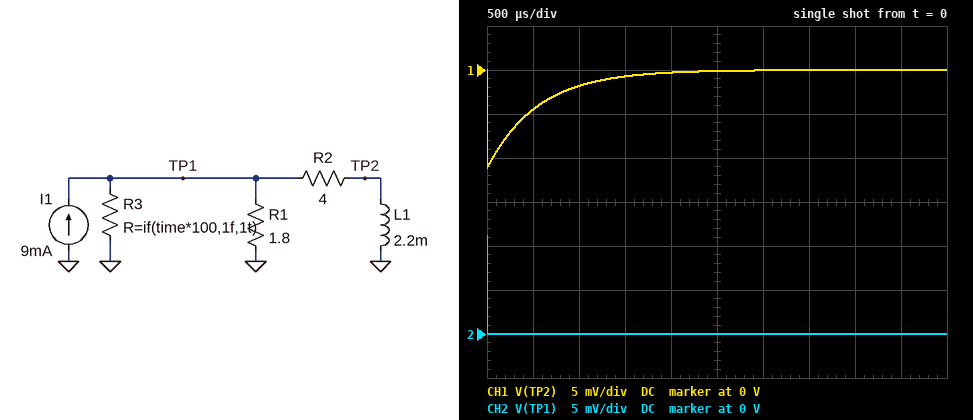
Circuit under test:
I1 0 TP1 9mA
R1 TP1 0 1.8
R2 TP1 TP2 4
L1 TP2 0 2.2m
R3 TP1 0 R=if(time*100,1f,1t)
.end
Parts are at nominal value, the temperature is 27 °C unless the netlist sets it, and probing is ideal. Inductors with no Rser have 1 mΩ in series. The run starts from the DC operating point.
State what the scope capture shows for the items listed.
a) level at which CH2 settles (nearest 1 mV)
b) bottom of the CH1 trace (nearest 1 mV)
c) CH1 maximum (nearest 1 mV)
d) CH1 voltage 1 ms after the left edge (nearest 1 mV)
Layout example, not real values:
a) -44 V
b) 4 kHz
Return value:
a) 0 V
b) -11 mV
c) 0 V
d) -2 mV
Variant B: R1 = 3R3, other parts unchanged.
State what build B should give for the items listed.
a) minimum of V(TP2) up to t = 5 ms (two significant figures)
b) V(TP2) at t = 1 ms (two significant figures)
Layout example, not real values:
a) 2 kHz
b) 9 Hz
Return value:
a) -16 mV
b) -2.6 mV
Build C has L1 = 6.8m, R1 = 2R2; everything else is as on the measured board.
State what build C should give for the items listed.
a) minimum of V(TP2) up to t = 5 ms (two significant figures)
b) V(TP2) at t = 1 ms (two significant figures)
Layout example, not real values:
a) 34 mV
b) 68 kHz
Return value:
a) -13 mV
b) -7.1 mV
